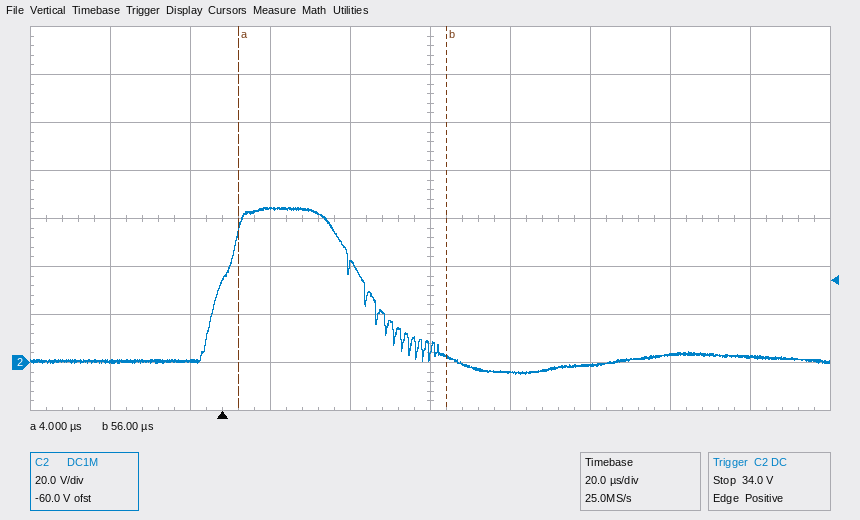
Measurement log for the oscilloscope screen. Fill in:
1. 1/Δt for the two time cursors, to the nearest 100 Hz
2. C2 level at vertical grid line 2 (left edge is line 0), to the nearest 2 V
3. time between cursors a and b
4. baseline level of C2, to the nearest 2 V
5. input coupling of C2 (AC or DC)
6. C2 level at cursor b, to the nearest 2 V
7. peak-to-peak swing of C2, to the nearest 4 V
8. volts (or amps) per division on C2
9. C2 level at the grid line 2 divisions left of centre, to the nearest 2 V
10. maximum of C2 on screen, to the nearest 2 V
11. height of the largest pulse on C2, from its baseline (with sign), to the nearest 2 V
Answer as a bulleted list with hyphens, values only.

- 19.2 kHz
- 0 V
- 52 µs
- 0 V
- DC
- 2 V
- 68 V
- 20 V
- 64 V
- 64 V
- +64 V
